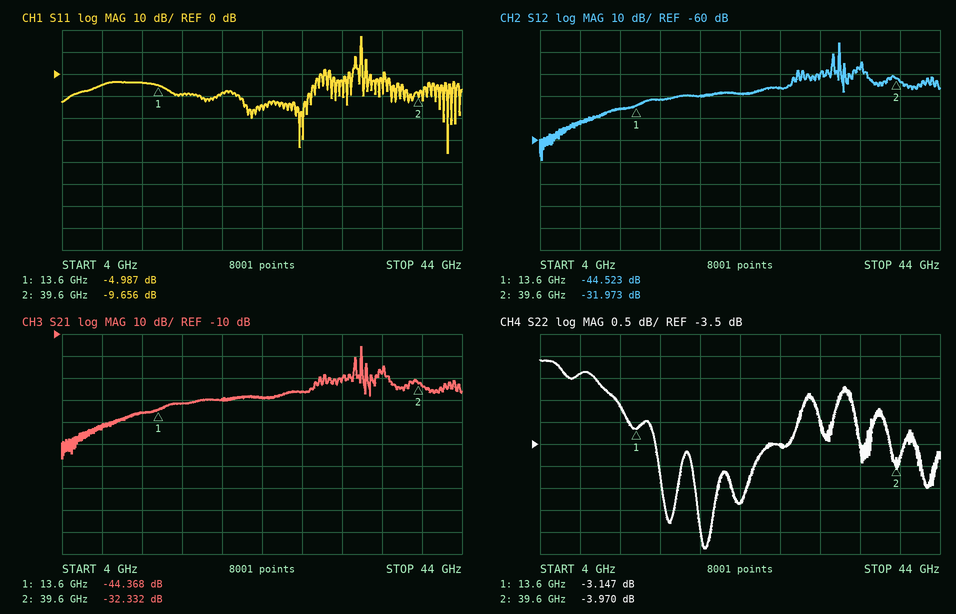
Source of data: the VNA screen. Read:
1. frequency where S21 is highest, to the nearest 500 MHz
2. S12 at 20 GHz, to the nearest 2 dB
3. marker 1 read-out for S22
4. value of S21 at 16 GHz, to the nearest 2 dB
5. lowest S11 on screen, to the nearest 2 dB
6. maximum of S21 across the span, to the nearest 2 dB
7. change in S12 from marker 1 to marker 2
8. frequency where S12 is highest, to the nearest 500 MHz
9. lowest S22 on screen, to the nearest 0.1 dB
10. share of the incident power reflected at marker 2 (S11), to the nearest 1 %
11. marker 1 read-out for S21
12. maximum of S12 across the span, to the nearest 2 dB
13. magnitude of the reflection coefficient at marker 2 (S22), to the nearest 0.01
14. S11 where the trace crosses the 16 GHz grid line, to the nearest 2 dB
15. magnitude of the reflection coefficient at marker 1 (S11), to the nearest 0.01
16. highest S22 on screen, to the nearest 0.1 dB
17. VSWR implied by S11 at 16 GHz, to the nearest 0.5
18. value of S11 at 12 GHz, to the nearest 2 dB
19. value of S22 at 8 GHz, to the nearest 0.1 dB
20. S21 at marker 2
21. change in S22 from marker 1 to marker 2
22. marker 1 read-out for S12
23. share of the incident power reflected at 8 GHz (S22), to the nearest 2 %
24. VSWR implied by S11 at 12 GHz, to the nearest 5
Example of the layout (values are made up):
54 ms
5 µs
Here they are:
34.0 GHz
-40 dB
-3.147 dB
-42 dB
-36 dB
-16 dB
12.550 dB
34.0 GHz
-5.9 dB
11 %
-44.368 dB
-16 dB
0.63
-10 dB
0.56
-1.6 dB
2.0
-4 dB
-1.9 dB
-32.332 dB
-0.823 dB
-44.523 dB
64 %
5
